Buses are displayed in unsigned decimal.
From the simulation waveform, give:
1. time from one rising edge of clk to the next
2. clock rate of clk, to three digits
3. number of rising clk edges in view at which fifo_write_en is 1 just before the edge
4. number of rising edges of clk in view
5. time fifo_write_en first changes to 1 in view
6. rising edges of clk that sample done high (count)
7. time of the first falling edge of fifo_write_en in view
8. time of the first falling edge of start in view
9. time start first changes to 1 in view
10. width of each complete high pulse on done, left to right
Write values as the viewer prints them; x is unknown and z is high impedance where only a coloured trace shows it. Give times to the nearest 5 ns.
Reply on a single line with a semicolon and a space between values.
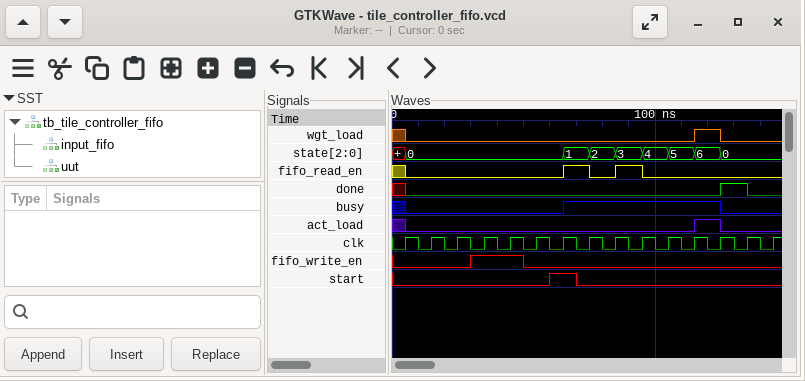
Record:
10 ns; 100 MHz; 2; 15; 30 ns; 1; 50 ns; 70 ns; 60 ns; 10 ns
